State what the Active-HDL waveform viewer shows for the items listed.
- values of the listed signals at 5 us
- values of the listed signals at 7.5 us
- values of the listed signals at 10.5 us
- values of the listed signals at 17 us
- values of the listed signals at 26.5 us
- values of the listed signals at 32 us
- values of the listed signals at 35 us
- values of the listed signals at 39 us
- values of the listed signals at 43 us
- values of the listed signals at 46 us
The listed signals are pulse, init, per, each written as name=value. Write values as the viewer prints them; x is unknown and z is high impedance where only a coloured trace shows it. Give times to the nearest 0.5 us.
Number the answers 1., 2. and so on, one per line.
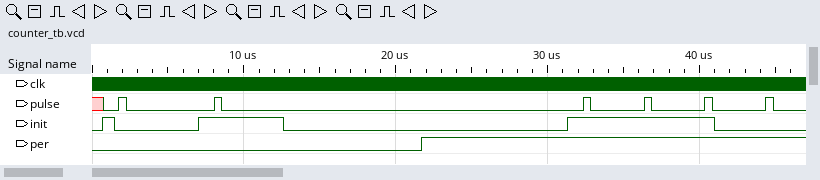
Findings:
1. pulse=0, init=0, per=0
2. pulse=0, init=1, per=0
3. pulse=0, init=1, per=0
4. pulse=0, init=0, per=0
5. pulse=0, init=0, per=1
6. pulse=0, init=1, per=1
7. pulse=0, init=1, per=1
8. pulse=0, init=1, per=1
9. pulse=0, init=0, per=1
10. pulse=0, init=0, per=1
